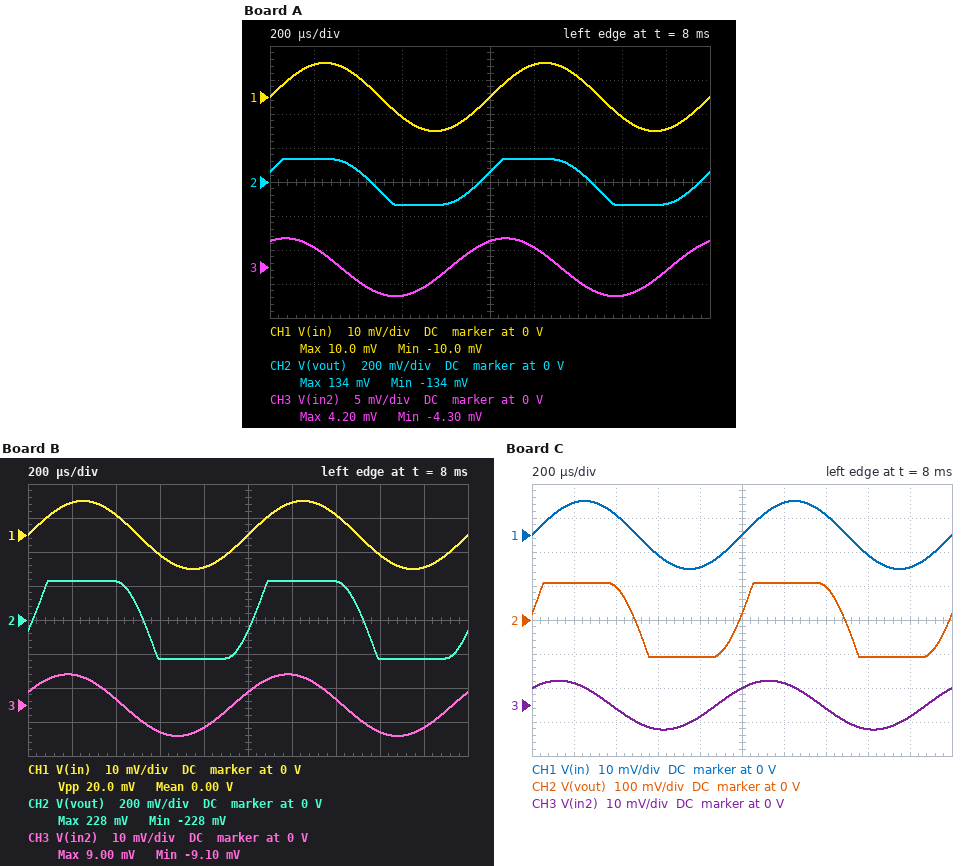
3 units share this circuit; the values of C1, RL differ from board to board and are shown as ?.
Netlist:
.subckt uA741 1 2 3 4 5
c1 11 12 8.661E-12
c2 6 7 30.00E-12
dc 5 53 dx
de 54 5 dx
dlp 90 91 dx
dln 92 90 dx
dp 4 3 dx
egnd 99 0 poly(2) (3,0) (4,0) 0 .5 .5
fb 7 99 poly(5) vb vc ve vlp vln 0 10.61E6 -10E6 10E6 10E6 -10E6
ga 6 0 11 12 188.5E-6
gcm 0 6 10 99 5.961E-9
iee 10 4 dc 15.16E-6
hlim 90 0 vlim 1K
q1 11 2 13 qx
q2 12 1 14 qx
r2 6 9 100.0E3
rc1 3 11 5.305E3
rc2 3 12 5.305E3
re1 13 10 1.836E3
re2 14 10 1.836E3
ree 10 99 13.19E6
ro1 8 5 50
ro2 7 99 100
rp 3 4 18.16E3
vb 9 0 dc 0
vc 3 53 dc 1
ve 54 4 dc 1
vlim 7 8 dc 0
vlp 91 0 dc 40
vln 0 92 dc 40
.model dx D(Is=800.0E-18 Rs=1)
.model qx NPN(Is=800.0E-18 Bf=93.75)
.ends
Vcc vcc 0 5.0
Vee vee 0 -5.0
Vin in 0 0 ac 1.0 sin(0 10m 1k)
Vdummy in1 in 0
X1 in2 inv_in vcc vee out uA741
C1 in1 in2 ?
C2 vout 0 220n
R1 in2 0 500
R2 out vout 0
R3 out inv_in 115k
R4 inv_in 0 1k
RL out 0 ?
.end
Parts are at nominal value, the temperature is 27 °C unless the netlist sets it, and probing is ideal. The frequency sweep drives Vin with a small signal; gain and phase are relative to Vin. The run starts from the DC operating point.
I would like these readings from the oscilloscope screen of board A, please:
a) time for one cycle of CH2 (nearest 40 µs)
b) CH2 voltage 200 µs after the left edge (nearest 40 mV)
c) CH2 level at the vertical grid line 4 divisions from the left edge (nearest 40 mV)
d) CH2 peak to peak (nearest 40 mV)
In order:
1.00 ms
120 mV
-120 mV
280 mV
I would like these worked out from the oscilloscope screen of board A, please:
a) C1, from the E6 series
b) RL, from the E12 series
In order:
150 nF
3.3 Ω
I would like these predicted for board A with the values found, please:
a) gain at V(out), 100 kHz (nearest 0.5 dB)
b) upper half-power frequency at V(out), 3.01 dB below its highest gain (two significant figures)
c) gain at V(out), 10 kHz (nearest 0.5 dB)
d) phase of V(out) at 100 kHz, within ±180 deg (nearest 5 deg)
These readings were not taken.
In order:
-5.0 dB
3.1 kHz
15.5 dB
-115 deg
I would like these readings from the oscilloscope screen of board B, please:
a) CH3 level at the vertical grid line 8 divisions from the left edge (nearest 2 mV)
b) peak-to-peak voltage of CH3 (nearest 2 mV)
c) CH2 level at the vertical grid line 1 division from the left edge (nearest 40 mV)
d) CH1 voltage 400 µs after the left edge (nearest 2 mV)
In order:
-8 mV
18 mV
240 mV
6 mV
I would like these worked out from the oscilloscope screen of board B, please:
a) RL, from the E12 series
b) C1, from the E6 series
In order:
5.6 Ω
680 nF
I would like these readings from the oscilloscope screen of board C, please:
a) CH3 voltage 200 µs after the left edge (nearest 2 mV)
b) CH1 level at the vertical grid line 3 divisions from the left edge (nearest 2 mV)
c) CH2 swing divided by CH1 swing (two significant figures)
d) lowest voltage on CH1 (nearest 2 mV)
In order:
6 mV
-6 mV
11
-10 mV
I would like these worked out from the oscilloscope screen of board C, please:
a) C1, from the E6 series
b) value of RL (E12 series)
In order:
330 nF
2.7 Ω
